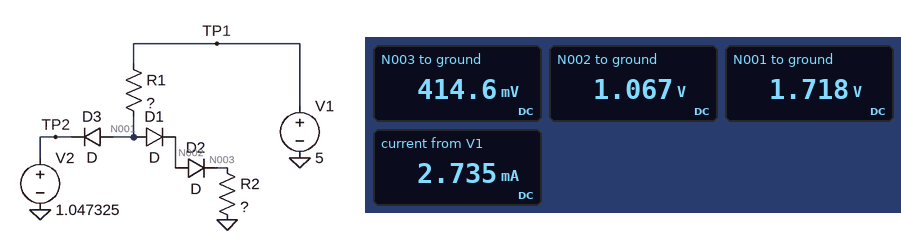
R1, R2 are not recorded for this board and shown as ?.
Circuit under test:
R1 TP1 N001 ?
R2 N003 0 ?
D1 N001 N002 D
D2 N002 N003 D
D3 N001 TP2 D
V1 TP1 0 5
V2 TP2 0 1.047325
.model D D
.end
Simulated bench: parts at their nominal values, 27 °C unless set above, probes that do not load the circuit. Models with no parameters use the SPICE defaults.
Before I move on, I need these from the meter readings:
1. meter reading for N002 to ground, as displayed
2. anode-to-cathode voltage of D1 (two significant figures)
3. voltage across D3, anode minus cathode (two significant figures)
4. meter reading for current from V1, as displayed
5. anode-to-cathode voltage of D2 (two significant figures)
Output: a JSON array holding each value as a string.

["1.067 V", "650 mV", "670 mV", "2.735 mA", "650 mV"]
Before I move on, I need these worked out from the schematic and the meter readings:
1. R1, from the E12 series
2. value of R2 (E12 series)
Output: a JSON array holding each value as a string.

["1.2 kΩ", "470 Ω"]
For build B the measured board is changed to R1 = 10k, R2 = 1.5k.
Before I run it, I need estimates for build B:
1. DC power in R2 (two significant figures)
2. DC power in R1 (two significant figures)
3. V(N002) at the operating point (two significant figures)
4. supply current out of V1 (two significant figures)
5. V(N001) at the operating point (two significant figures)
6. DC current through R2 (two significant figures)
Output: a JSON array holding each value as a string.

["100 µW", "1.1 mW", "1.0 V", "340 µA", "1.6 V", "260 µA"]
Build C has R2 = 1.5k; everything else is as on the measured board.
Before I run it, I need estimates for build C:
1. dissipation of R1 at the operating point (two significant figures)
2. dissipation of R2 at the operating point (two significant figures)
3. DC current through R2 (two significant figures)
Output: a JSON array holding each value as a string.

["8.9 mW", "150 µW", "320 µA"]
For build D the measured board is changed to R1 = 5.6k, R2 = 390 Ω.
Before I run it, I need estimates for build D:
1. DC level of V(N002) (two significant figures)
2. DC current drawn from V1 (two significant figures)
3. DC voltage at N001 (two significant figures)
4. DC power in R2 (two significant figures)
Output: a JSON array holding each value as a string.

["880 mV", "620 µA", "1.5 V", "150 µW"]
